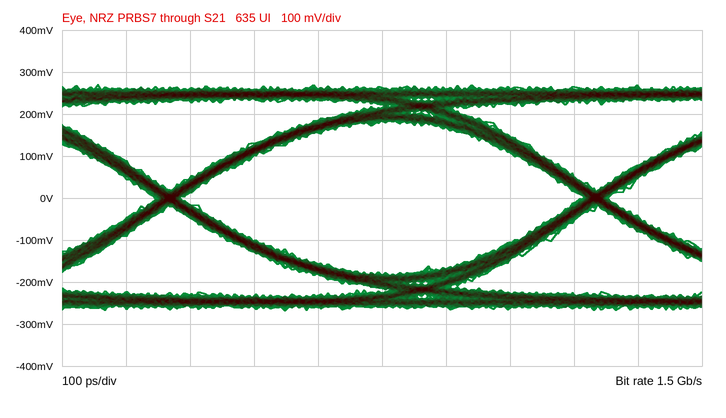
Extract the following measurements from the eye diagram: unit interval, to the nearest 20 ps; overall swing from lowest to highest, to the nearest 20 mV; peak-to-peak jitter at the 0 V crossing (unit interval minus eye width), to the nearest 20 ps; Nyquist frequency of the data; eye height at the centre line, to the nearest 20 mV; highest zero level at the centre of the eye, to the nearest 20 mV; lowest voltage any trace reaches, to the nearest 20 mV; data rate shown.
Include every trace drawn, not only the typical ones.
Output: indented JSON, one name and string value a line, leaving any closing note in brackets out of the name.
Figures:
{
  "unit interval, to the nearest 20 ps": "660 ps",
  "overall swing from lowest to highest, to the nearest 20 mV": "540 mV",
  "peak-to-peak jitter at the 0 V crossing (unit interval minus eye width), to the nearest 20 ps": "40 ps",
  "Nyquist frequency of the data": "750 MHz",
  "eye height at the centre line, to the nearest 20 mV": "360 mV",
  "highest zero level at the centre of the eye, to the nearest 20 mV": "-180 mV",
  "lowest voltage any trace reaches, to the nearest 20 mV": "-260 mV",
  "data rate shown": "1.5 Gb/s"
}
